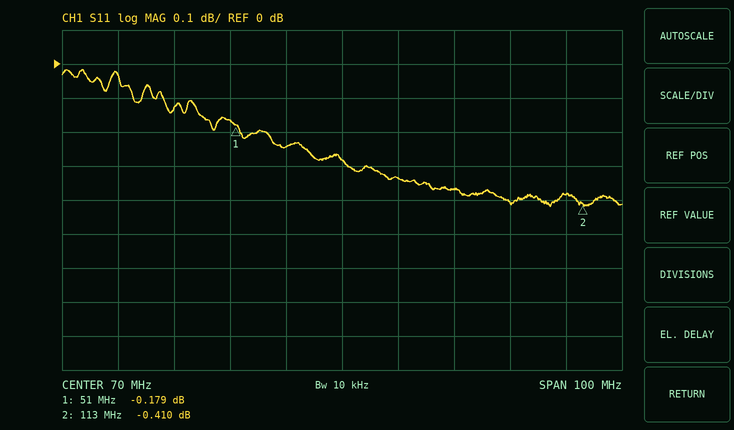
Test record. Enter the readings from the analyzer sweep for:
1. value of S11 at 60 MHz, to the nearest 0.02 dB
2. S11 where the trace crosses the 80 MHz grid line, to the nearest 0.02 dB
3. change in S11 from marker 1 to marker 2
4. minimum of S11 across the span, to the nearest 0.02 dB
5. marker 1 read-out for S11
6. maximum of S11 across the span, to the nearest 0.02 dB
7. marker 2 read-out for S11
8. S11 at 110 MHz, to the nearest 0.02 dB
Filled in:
-0.24 dB
-0.34 dB
-0.231 dB
-0.42 dB
-0.179 dB
-0.02 dB
-0.410 dB
-0.38 dB
